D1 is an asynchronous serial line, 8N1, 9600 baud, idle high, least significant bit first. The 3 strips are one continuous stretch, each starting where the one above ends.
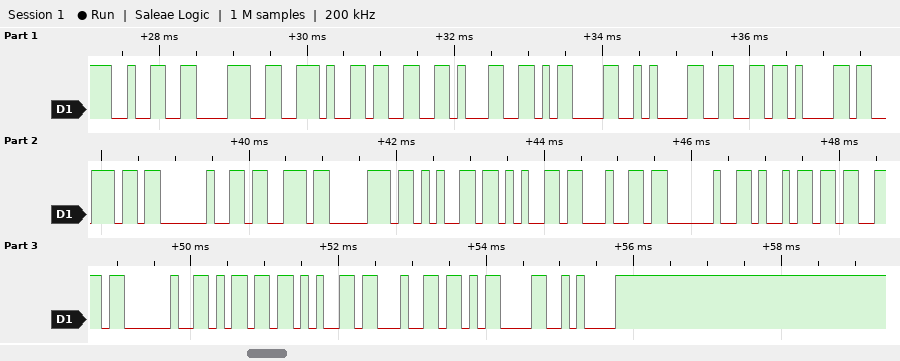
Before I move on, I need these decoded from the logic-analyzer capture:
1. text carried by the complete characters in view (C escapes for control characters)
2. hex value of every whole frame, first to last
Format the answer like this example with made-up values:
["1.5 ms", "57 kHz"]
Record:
["\"28.31\\r\\nfan speed is med\\r\\n\"", "0x32 0x38 0x2E 0x33 0x31 0x0D 0x0A 0x66 0x61 0x6E 0x20 0x73 0x70 0x65 0x65 0x64 0x20 0x69 0x73 0x20 0x6D 0x65 0x64 0x0D 0x0A"]
